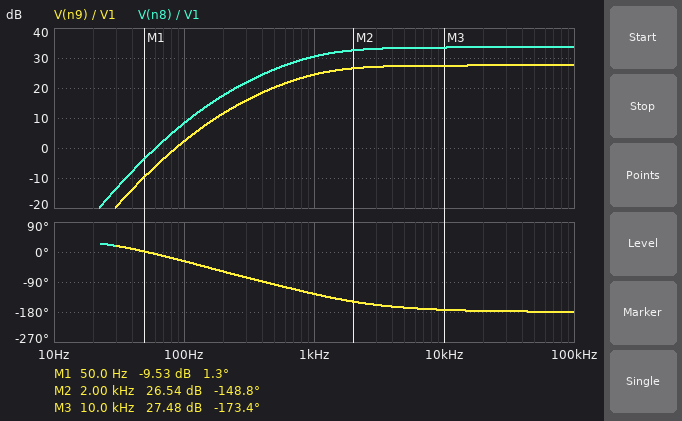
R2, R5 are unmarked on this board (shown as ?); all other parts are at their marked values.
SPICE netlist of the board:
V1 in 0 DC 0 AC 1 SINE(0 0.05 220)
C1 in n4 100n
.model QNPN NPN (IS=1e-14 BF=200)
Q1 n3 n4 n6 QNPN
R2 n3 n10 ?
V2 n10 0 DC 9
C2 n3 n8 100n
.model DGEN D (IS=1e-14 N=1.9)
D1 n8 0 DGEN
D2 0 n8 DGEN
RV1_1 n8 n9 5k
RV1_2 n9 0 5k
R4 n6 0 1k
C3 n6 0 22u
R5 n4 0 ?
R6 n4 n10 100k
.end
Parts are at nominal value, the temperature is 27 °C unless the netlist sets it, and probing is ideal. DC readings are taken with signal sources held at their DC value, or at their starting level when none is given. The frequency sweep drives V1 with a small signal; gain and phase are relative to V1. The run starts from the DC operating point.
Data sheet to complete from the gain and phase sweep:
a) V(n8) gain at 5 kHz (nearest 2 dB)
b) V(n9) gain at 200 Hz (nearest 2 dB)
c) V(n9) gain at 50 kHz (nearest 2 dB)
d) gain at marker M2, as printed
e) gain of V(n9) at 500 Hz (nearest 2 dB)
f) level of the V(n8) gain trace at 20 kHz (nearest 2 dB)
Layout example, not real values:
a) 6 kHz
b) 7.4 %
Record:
a) 34 dB
b) 12 dB
c) 28 dB
d) 26.54 dB
e) 20 dB
f) 34 dB
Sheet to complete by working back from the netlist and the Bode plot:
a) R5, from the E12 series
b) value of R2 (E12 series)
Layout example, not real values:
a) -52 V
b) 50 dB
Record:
a) 39 kΩ
b) 820 Ω
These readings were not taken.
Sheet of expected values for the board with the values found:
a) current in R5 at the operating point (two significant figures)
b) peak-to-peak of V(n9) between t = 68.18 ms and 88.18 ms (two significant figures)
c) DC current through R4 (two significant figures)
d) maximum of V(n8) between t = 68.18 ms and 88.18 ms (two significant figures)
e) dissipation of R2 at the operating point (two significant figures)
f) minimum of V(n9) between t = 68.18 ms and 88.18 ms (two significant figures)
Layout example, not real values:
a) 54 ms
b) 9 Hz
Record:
a) 59 µA
b) 420 mV
c) 1.6 mA
d) 400 mV
e) 2.2 mW
f) -220 mV
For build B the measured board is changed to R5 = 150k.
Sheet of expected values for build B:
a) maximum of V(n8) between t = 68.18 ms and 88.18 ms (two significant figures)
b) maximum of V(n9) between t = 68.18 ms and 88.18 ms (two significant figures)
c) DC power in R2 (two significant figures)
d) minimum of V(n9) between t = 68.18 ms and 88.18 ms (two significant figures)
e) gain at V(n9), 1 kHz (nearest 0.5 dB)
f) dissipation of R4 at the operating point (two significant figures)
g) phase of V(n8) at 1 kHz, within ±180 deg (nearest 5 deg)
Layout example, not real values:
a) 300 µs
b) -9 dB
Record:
a) 440 mV
b) 220 mV
c) 11 mW
d) -230 mV
e) 27.0 dB
f) 13 mW
g) -105 deg
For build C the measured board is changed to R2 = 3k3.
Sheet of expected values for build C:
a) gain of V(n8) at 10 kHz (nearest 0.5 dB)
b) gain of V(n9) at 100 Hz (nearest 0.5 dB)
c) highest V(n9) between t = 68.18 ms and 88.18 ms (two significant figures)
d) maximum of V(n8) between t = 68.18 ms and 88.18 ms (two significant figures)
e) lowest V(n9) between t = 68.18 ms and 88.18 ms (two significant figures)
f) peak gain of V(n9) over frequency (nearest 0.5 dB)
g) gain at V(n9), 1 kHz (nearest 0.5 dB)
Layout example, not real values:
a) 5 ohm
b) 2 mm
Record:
a) 44.0 dB
b) 13.5 dB
c) 560 mV
d) 1.1 V
e) -570 mV
f) 38.0 dB
g) 35.0 dB
